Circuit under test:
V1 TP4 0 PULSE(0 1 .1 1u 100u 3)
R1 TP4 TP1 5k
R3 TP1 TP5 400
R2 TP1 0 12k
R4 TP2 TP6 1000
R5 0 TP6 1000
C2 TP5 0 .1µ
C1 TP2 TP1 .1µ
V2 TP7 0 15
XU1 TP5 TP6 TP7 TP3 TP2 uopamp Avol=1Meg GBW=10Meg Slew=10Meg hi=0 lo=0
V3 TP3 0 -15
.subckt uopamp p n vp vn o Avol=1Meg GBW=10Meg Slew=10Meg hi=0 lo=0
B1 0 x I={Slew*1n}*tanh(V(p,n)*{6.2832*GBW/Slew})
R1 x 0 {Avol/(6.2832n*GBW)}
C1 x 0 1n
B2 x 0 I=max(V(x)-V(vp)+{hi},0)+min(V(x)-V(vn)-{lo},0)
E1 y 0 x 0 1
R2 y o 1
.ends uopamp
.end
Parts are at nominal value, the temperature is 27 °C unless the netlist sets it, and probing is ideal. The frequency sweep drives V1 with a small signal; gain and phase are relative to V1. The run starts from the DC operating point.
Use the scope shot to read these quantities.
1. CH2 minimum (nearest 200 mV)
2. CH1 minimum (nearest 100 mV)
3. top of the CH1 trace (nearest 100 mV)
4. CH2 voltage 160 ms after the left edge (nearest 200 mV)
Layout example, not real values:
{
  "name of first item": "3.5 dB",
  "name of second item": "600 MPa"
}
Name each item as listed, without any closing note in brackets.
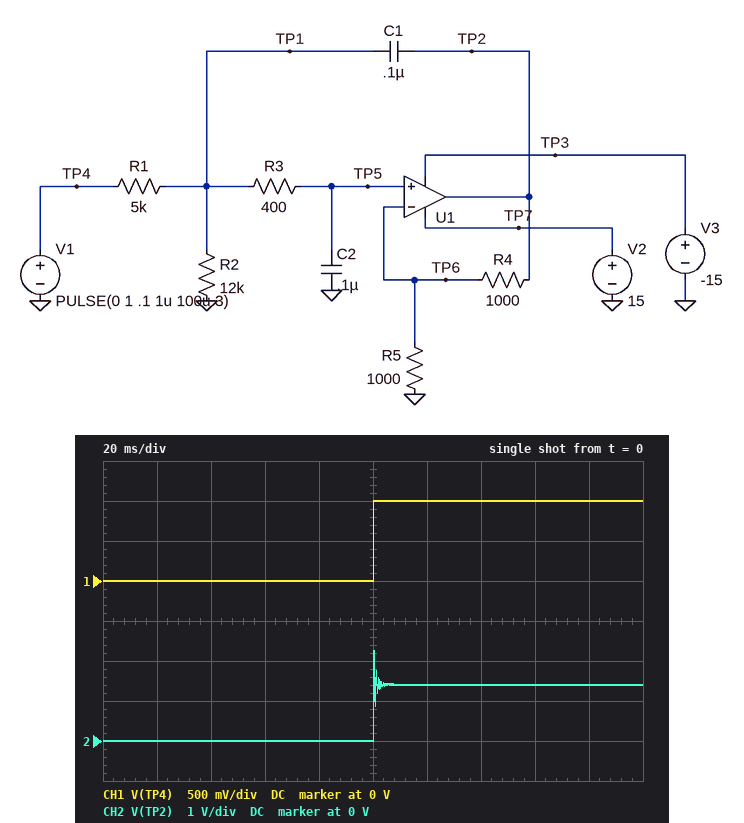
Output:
{
  "CH2 minimum": "0 V",
  "CH1 minimum": "0 V",
  "top of the CH1 trace": "1.0 V",
  "CH2 voltage 160 ms after the left edge": "1.4 V"
}
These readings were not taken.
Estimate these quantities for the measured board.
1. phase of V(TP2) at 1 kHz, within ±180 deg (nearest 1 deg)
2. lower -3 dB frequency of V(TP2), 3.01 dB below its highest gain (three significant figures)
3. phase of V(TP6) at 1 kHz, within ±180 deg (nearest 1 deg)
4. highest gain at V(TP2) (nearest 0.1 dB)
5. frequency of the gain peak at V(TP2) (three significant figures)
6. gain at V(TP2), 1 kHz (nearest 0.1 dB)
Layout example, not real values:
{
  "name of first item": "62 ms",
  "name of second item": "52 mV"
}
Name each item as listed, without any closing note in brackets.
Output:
{
  "phase of V(TP2) at 1 kHz, within ±180 deg": "-30 deg",
  "lower -3 dB frequency of V(TP2), 3.01 dB below its highest gain": "1.05 kHz",
  "phase of V(TP6) at 1 kHz, within ±180 deg": "-30 deg",
  "highest gain at V(TP2)": "12.6 dB",
  "frequency of the gain peak at V(TP2)": "1.30 kHz",
  "gain at V(TP2), 1 kHz": "8.9 dB"
}
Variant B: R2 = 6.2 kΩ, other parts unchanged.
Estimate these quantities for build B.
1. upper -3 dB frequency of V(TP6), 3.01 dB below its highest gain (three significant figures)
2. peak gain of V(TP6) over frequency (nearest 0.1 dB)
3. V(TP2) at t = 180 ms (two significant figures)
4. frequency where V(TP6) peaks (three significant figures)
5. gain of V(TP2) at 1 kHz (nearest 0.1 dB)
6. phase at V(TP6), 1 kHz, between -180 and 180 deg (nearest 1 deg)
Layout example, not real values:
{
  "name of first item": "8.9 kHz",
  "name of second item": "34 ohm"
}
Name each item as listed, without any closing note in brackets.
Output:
{
  "upper -3 dB frequency of V(TP6), 3.01 dB below its highest gain": "1.72 kHz",
  "peak gain of V(TP6) over frequency": "3.4 dB",
  "V(TP2) at t = 180 ms": "1.1 V",
  "frequency where V(TP6) peaks": "1.46 kHz",
  "gain of V(TP2) at 1 kHz": "5.1 dB",
  "phase at V(TP6), 1 kHz, between -180 and 180 deg": "-24 deg"
}
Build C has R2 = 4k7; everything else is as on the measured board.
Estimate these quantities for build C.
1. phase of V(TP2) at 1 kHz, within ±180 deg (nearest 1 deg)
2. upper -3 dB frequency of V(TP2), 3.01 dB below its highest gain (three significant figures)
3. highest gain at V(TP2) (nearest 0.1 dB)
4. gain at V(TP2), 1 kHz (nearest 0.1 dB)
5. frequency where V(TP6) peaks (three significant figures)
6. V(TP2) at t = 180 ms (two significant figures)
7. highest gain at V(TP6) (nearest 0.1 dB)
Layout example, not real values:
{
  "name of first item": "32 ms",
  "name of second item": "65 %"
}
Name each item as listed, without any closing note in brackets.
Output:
{
  "phase of V(TP2) at 1 kHz, within ±180 deg": "-22 deg",
  "upper -3 dB frequency of V(TP2), 3.01 dB below its highest gain": "1.85 kHz",
  "highest gain at V(TP2)": "7.7 dB",
  "gain at V(TP2), 1 kHz": "3.3 dB",
  "frequency where V(TP6) peaks": "1.55 kHz",
  "V(TP2) at t = 180 ms": "970 mV",
  "highest gain at V(TP6)": "1.7 dB"
}
